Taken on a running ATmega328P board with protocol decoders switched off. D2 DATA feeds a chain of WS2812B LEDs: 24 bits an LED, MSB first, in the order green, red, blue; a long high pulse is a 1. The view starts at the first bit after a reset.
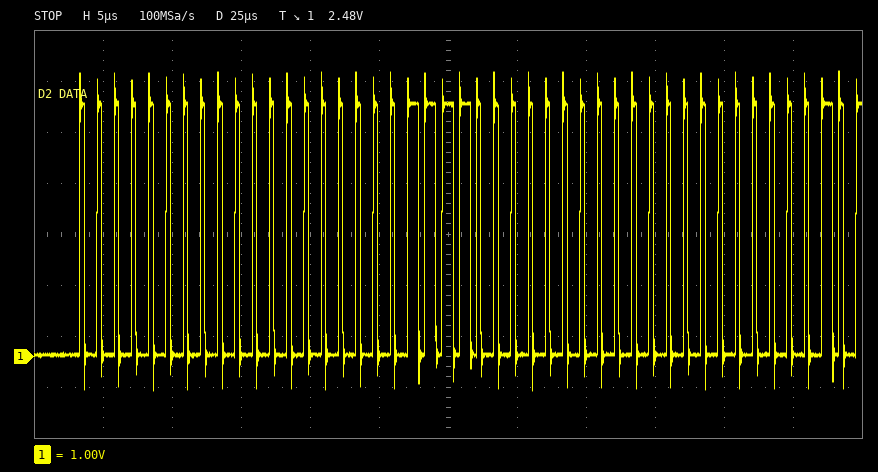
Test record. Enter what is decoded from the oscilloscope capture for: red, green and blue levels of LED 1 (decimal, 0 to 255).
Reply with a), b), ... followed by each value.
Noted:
a) 0, 0, 30
